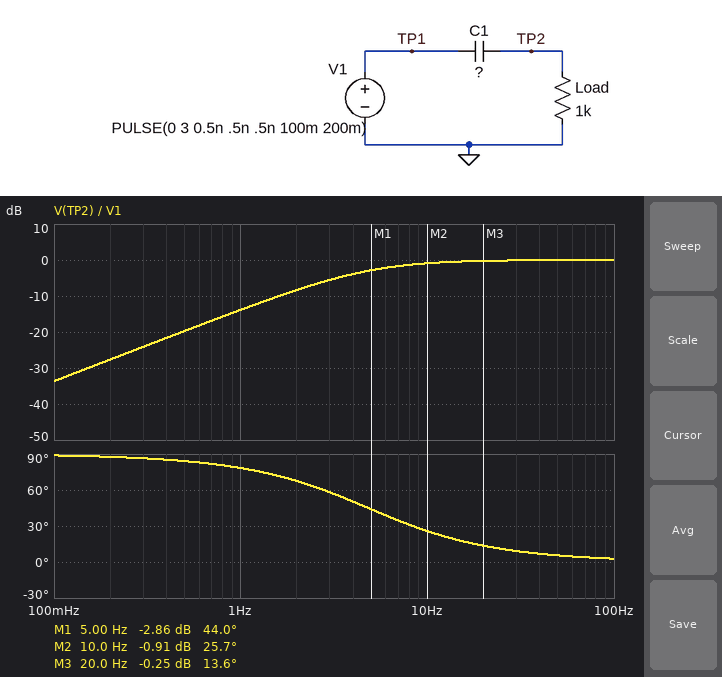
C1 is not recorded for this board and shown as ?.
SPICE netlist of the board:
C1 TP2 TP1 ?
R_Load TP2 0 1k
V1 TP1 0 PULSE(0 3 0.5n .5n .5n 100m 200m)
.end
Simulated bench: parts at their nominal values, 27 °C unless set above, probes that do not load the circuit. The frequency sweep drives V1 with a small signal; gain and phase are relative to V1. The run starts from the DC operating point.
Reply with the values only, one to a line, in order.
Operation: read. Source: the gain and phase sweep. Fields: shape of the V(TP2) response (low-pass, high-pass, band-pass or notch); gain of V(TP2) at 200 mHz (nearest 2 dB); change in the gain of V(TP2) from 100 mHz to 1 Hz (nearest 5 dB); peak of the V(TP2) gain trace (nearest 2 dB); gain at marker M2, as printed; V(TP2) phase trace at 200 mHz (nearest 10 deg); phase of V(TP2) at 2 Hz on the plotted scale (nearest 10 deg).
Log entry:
high-pass
-28 dB
20 dB
0 dB
-0.91 dB
90 deg
70 deg
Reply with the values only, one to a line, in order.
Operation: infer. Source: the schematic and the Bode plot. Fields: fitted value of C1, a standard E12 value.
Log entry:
33 µF
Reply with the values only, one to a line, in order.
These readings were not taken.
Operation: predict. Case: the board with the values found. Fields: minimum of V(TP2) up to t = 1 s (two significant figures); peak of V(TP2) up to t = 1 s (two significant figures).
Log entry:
-2.9 V
3.0 V
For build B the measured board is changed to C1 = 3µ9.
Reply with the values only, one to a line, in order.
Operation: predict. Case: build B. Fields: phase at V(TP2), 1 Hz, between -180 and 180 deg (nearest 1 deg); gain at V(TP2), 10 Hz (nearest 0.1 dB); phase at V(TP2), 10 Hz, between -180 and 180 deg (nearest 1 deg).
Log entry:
89 deg
-12.5 dB
76 deg
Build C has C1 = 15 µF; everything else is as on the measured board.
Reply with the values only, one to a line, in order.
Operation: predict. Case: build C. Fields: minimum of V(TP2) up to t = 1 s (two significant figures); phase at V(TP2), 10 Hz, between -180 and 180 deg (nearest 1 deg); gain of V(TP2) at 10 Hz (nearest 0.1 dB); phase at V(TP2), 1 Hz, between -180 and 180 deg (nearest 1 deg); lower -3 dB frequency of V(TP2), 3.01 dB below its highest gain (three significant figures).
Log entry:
-3.0 V
47 deg
-3.3 dB
85 deg
10.6 Hz
